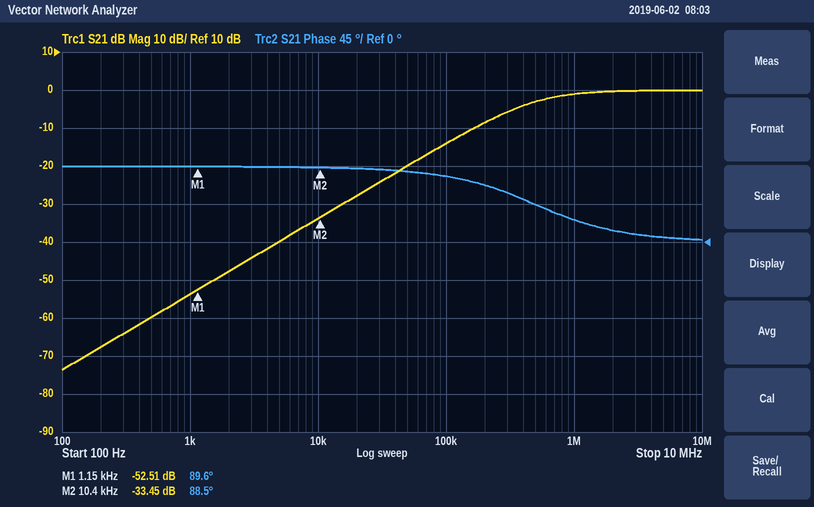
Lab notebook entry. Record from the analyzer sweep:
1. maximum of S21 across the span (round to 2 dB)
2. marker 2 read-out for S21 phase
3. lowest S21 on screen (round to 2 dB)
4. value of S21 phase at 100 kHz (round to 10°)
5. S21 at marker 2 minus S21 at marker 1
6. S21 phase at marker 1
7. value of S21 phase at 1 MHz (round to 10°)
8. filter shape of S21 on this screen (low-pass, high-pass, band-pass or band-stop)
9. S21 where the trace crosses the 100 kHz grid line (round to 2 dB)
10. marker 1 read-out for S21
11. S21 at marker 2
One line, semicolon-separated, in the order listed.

0 dB; 88.5°; -74 dB; 80°; 19.06 dB; 89.6°; 30°; high-pass; -14 dB; -52.51 dB; -33.45 dB
